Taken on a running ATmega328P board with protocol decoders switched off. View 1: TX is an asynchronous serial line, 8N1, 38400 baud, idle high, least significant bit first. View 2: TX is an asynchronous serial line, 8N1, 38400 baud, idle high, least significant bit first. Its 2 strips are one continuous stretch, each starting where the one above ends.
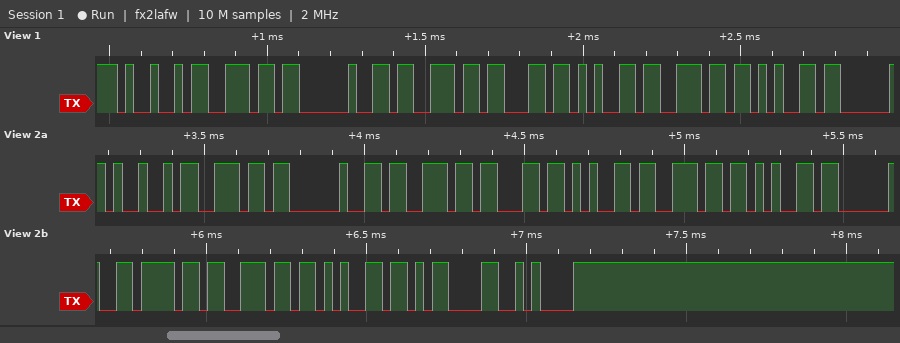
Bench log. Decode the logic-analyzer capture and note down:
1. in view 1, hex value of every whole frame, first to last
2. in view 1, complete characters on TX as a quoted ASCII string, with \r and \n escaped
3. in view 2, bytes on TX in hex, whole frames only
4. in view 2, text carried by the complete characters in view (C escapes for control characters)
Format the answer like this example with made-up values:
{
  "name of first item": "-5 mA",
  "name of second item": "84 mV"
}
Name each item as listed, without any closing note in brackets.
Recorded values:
{
  "in view 1, hex value of every whole frame, first to last": "49 6E 20 73 63 65 6E 65",
  "in view 1, complete characters on TX as a quoted ASCII string, with \\r and \\n escaped": "\"In scene\"",
  "in view 2, bytes on TX in hex, whole frames only": "49 6E 20 73 63 65 6E 65 20 6F 6E 65 0D 0A",
  "in view 2, text carried by the complete characters in view": "\"In scene one\\r\\n\""
}
